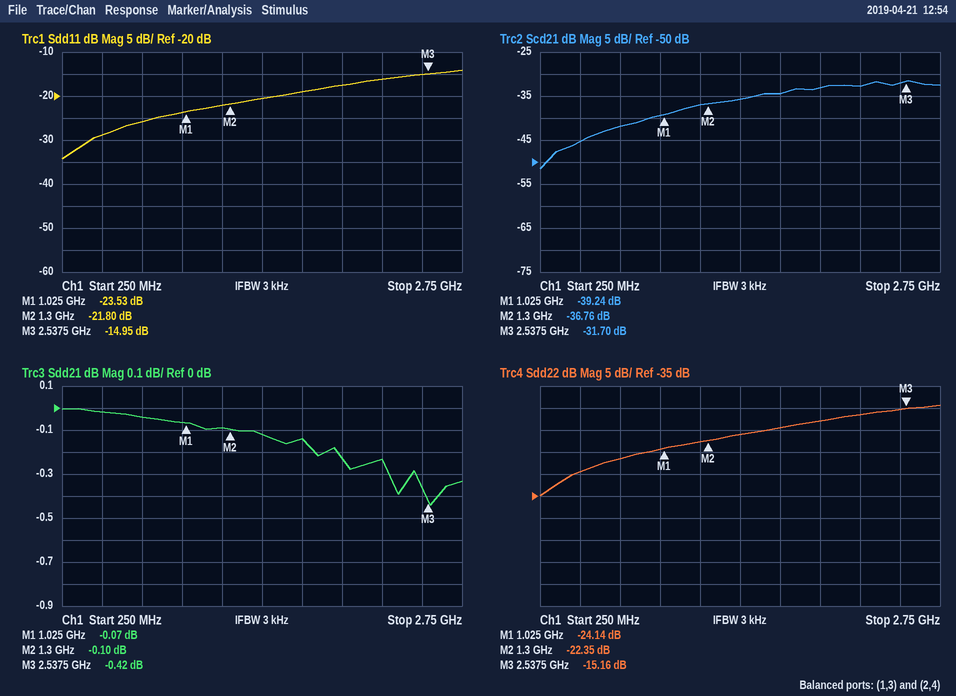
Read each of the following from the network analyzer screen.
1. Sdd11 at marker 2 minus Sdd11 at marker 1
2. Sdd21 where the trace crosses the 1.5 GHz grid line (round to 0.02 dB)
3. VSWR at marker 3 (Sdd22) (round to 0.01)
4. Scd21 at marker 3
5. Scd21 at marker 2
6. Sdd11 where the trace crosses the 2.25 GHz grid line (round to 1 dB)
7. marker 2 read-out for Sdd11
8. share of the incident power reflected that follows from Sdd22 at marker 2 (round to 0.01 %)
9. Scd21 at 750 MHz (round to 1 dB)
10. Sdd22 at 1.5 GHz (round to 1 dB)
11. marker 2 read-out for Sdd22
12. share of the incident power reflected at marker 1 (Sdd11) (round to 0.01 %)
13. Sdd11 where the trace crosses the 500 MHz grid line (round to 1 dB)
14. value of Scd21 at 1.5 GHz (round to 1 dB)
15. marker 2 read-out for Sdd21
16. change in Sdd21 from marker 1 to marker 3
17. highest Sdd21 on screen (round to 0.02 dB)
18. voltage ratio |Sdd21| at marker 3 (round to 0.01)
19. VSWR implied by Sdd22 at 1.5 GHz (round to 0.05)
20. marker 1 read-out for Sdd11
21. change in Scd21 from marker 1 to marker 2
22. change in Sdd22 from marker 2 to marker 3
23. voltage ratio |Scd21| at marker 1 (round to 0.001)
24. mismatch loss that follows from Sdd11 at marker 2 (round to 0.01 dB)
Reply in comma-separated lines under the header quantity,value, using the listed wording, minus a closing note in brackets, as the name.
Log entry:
quantity,value
Sdd11 at marker 2 minus Sdd11 at marker 1,1.73 dB
Sdd21 where the trace crosses the 1.5 GHz grid line,-0.12 dB
VSWR at marker 3 (Sdd22),1.42
Scd21 at marker 3,-31.70 dB
Scd21 at marker 2,-36.76 dB
Sdd11 where the trace crosses the 2.25 GHz grid line,-16 dB
marker 2 read-out for Sdd11,-21.80 dB
share of the incident power reflected that follows from Sdd22 at marker 2,0.58 %
Scd21 at 750 MHz,-42 dB
Sdd22 at 1.5 GHz,-21 dB
marker 2 read-out for Sdd22,-22.35 dB
share of the incident power reflected at marker 1 (Sdd11),0.44 %
Sdd11 where the trace crosses the 500 MHz grid line,-29 dB
value of Scd21 at 1.5 GHz,-36 dB
marker 2 read-out for Sdd21,-0.10 dB
change in Sdd21 from marker 1 to marker 3,-0.35 dB
highest Sdd21 on screen,0.00 dB
voltage ratio |Sdd21| at marker 3,0.95
VSWR implied by Sdd22 at 1.5 GHz,1.20
marker 1 read-out for Sdd11,-23.53 dB
change in Scd21 from marker 1 to marker 2,2.48 dB
change in Sdd22 from marker 2 to marker 3,7.19 dB
voltage ratio |Scd21| at marker 1,0.011
mismatch loss that follows from Sdd11 at marker 2,0.03 dB
